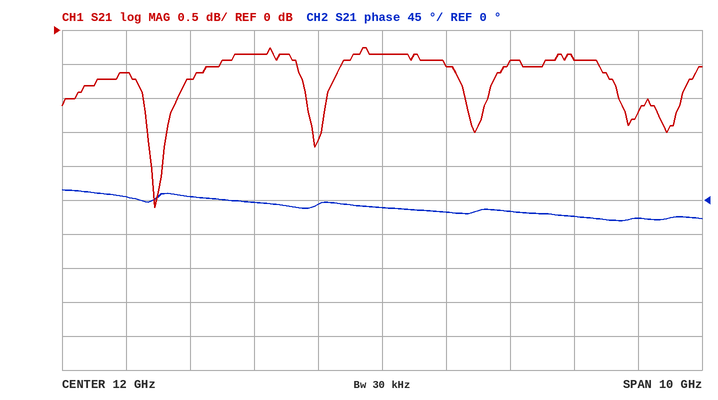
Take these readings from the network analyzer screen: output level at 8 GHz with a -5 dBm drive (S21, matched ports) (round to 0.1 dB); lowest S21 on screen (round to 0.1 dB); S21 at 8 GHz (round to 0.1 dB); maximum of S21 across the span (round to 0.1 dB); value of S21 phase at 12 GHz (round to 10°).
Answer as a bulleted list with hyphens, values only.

- -5.6 dBm
- -2.6 dB
- -0.6 dB
- -0.3 dB
- -10°
